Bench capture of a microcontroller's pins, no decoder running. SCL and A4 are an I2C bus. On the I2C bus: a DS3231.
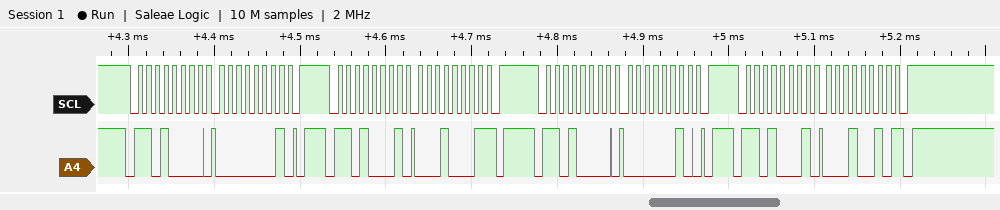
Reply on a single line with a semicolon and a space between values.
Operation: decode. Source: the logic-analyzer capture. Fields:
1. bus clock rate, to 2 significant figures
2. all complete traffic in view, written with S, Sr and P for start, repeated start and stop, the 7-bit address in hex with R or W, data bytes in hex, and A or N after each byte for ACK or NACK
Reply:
100 kHz; S 68W A 01 A P S 68R A 11 N P S 68W A 02 A P S 68R A 12 N P
